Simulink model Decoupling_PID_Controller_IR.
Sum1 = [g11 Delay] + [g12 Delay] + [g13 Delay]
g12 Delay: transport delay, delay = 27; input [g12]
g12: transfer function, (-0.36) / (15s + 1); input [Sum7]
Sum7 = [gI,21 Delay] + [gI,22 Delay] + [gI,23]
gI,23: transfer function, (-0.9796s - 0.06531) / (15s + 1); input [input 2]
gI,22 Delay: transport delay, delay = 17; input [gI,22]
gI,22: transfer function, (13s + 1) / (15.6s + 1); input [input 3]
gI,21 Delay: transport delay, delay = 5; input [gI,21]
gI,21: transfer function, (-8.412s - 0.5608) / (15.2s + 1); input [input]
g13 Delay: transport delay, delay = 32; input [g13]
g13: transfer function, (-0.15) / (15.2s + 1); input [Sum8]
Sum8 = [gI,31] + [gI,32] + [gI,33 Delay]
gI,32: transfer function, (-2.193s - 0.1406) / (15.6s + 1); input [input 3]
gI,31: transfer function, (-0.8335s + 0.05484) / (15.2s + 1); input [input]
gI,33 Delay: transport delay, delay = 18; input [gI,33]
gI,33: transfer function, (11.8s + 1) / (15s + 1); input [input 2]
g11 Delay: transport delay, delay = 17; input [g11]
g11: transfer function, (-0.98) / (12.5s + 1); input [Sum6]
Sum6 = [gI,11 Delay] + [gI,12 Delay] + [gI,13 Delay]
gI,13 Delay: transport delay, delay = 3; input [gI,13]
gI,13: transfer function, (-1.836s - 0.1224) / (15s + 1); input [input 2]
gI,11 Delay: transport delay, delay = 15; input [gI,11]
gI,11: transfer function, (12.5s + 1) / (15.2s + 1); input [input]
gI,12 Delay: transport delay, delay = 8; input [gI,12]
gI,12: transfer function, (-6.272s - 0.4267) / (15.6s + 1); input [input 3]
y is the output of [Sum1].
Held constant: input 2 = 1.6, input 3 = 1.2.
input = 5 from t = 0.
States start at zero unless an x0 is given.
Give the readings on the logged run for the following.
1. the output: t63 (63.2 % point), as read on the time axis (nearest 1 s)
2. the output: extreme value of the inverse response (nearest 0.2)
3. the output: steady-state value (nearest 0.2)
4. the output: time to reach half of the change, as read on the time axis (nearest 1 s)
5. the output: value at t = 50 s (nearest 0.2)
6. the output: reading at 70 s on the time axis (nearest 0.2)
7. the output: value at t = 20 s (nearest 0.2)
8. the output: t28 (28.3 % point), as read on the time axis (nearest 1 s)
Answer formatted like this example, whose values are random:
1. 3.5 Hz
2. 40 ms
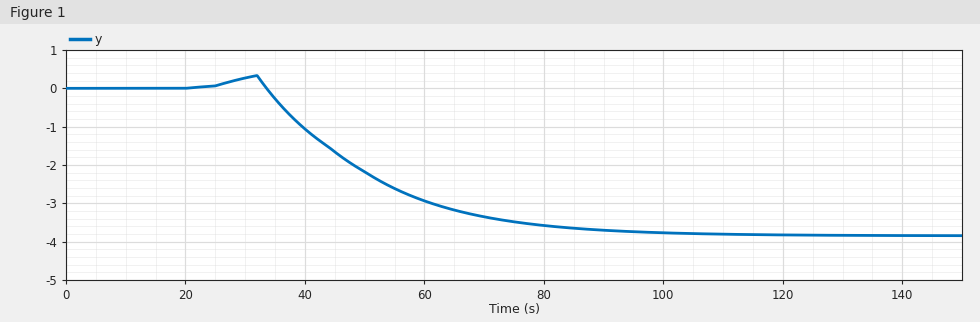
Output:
1. 53 s
2. 0.4
3. -3.8
4. 47 s
5. -2.2
6. -3.4
7. 0.0
8. 40 s
